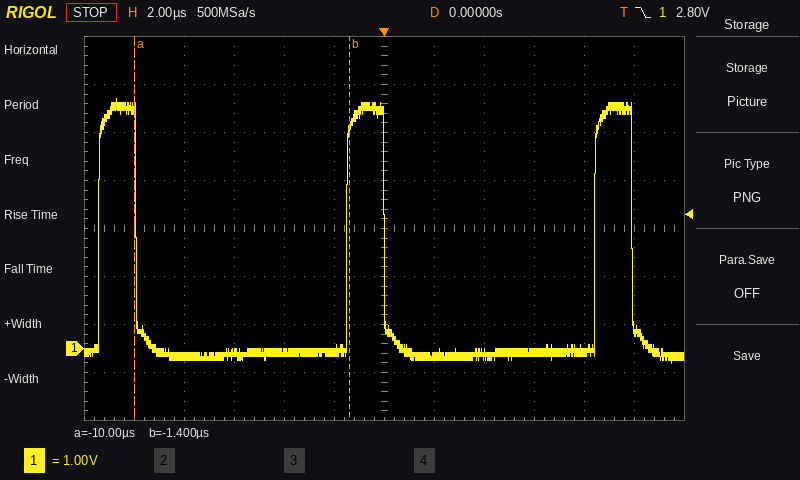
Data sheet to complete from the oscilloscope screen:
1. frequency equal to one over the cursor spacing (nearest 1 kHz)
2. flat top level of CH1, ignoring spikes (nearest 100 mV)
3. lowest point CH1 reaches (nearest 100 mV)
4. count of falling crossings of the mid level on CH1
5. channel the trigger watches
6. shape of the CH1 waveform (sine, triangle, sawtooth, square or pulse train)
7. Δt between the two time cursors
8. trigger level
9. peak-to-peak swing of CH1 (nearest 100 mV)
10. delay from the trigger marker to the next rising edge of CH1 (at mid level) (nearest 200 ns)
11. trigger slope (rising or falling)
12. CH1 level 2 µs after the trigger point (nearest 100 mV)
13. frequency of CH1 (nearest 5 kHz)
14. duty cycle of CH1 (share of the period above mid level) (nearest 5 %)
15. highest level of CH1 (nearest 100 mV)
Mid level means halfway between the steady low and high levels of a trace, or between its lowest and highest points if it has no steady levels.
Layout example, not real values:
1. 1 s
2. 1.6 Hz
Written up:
1. 116 kHz
2. 5.0 V
3. -300 mV
4. 3
5. CH1
6. pulse train
7. 8.6 µs
8. 2.80 V
9. 5.5 V
10. 8.4 µs
11. falling
12. -200 mV
13. 100 kHz
14. 15 %
15. 5.2 V
